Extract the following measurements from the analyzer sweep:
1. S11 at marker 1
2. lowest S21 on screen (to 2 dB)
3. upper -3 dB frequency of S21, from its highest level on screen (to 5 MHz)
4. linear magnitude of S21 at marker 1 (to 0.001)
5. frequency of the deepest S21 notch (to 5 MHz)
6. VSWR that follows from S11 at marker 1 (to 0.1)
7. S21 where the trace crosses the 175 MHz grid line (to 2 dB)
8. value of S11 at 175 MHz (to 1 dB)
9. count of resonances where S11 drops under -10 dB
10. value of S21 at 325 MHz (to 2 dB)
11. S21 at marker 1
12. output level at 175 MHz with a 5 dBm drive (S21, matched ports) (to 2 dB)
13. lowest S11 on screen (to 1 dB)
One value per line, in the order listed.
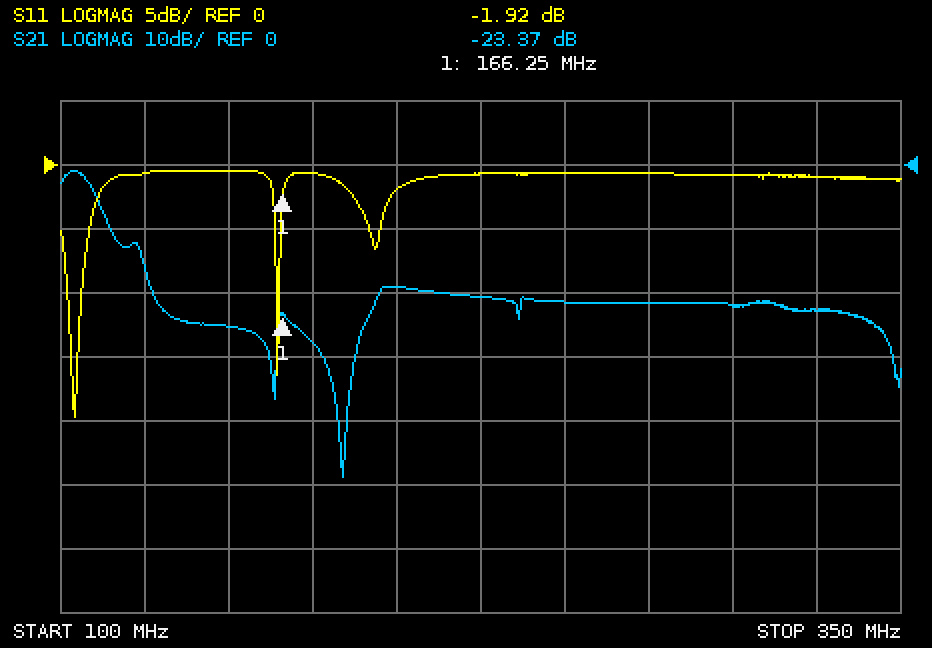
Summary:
-1.92 dB
-48 dB
110 MHz
0.068
185 MHz
9.1
-28 dB
-1 dB
2
-22 dB
-23.37 dB
-22 dBm
-20 dB
